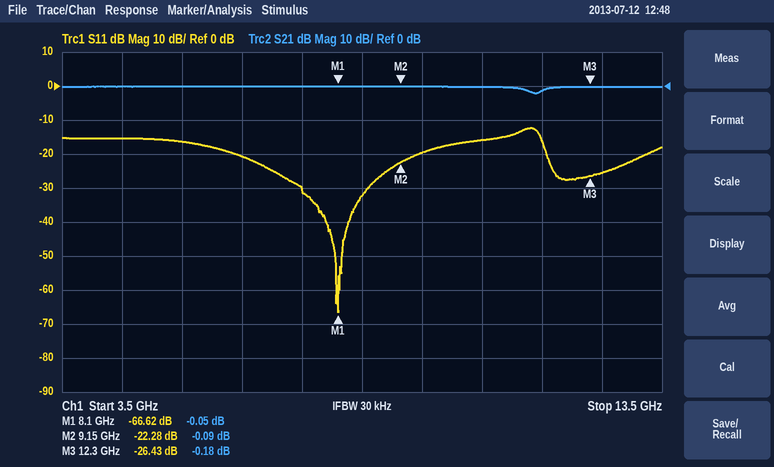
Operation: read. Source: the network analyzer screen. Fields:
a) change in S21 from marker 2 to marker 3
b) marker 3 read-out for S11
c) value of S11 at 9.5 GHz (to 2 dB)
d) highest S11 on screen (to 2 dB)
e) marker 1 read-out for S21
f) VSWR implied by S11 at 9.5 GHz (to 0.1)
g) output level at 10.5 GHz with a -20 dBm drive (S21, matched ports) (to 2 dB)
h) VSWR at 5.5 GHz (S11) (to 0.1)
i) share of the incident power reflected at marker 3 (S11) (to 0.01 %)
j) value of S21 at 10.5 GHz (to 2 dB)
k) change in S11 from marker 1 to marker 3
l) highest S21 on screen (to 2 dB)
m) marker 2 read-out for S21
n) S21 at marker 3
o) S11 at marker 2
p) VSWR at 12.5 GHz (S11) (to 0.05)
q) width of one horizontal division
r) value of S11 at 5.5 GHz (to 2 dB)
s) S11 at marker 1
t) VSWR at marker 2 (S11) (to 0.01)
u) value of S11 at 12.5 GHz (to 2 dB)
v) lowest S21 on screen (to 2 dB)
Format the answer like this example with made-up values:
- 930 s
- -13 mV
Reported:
- -0.09 dB
- -26.43 dB
- -20 dB
- -12 dB
- -0.05 dB
- 1.2
- -20 dBm
- 1.4
- 0.23 %
- 0 dB
- 40.19 dB
- 0 dB
- -0.09 dB
- -0.18 dB
- -22.28 dB
- 1.10
- 1 GHz
- -16 dB
- -66.62 dB
- 1.17
- -26 dB
- -2 dB
